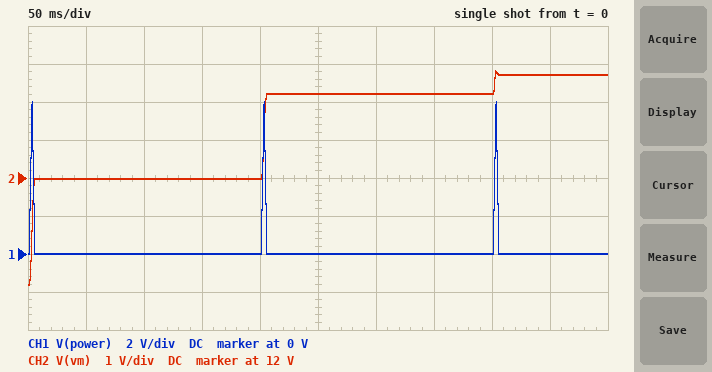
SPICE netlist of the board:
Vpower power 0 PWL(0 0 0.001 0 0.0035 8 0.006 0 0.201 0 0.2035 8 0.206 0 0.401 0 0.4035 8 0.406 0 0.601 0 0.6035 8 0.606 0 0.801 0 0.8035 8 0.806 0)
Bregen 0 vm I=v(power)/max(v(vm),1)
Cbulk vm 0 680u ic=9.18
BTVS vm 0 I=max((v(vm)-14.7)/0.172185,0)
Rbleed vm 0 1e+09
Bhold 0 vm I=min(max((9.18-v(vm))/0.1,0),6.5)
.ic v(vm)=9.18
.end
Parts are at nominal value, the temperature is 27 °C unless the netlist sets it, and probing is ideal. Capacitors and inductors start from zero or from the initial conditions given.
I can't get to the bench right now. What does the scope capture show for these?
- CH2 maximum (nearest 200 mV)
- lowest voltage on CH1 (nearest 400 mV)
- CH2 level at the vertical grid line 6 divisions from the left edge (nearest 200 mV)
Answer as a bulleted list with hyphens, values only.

- 14.8 V
- 0 V
- 14.2 V
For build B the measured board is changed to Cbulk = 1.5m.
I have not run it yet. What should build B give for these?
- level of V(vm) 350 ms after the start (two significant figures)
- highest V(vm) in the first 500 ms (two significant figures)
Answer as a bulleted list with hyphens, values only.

- 12 V
- 13 V
